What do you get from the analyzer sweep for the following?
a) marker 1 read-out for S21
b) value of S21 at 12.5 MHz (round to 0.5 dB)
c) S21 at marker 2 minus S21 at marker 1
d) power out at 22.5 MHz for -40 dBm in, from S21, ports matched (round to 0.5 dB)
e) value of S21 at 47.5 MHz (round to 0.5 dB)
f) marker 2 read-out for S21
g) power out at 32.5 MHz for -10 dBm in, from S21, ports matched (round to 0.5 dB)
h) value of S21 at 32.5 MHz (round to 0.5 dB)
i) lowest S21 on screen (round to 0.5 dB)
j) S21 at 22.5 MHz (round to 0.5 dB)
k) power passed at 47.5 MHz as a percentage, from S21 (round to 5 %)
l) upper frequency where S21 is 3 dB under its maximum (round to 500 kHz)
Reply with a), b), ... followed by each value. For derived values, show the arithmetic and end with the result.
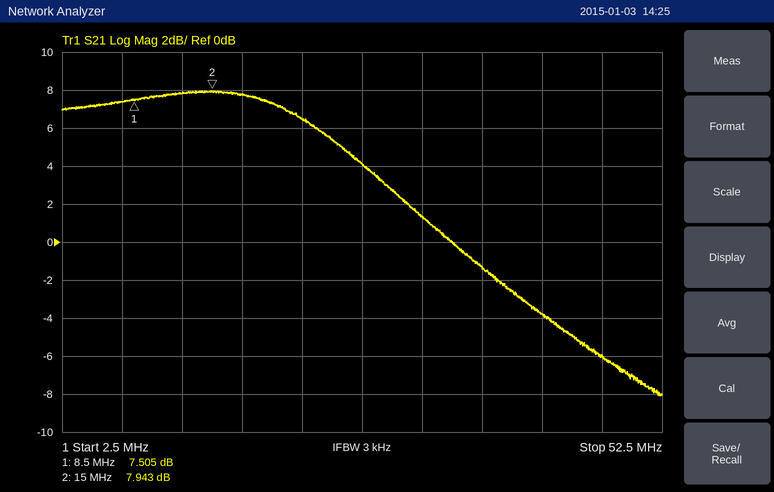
a) 7.505 dB
b) 8.0 dB
c) 7.943 − (7.505) = 0.438 dB
d) -40 dBm + (6.5 dB) = -33.5 dBm
e) -6.0 dB
f) 7.943 dB
g) -10 dBm + (1.5 dB) = -8.5 dBm
h) 1.5 dB
i) -8.0 dB
j) 6.5 dB
k) 10^(-6/10) ≈ 25 %
l) 26.0 MHz
